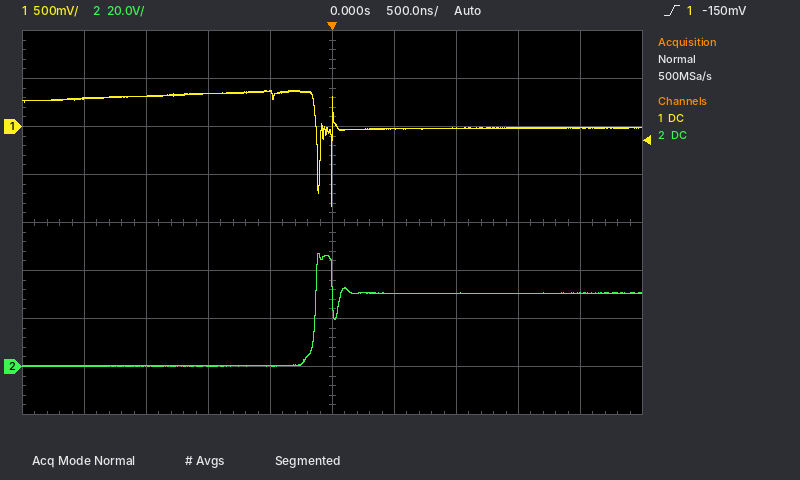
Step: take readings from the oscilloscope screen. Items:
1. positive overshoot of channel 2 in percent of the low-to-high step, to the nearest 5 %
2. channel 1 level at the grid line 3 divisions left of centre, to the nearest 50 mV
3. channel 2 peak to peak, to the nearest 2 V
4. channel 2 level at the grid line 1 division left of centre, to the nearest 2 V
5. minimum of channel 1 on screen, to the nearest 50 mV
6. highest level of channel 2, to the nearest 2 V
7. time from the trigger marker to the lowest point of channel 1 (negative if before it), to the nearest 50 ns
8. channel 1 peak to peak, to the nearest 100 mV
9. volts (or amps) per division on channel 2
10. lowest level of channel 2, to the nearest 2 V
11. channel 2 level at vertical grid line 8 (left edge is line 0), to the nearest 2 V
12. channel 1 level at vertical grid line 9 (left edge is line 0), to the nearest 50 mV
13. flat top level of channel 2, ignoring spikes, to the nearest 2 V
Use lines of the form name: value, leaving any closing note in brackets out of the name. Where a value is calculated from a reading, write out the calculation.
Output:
positive overshoot of channel 2 in percent of the low-to-high step, to the nearest 5 %: 55 %
channel 1 level at the grid line 3 divisions left of centre, to the nearest 50 mV: 300 mV
channel 2 peak to peak, to the nearest 2 V: 48 V − (0 V) = 48 V
channel 2 level at the grid line 1 division left of centre, to the nearest 2 V: 0 V
minimum of channel 1 on screen, to the nearest 50 mV: -850 mV
highest level of channel 2, to the nearest 2 V: 48 V
time from the trigger marker to the lowest point of channel 1 (negative if before it), to the nearest 50 ns: 0 ns
channel 1 peak to peak, to the nearest 100 mV: 1.20 V
volts (or amps) per division on channel 2: 20 V
lowest level of channel 2, to the nearest 2 V: 0 V
channel 2 level at vertical grid line 8 (left edge is line 0), to the nearest 2 V: 30 V
channel 1 level at vertical grid line 9 (left edge is line 0), to the nearest 50 mV: 0 mV
flat top level of channel 2, ignoring spikes, to the nearest 2 V: 30 V
